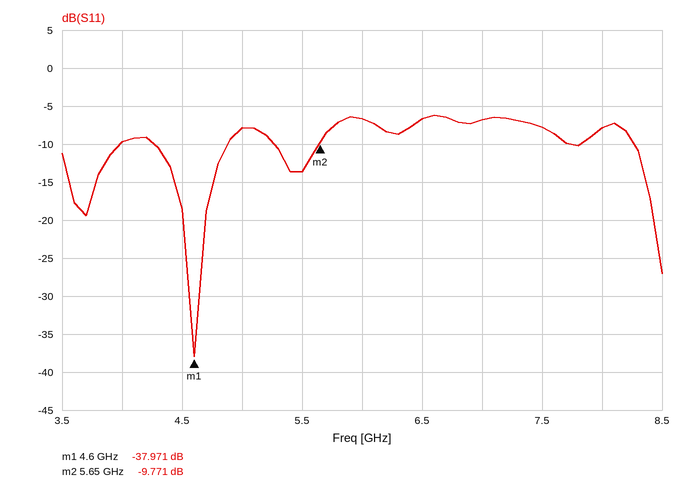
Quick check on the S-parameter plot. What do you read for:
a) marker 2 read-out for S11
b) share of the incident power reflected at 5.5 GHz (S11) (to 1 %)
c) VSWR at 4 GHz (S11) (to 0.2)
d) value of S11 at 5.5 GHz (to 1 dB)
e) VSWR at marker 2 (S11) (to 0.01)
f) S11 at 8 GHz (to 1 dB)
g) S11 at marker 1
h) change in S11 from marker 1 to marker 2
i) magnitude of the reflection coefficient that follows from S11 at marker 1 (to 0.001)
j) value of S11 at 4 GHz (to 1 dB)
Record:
-9.771 dB
4 %
2.0
-14 dB
1.96
-8 dB
-37.971 dB
28.200 dB
0.013
-10 dB
